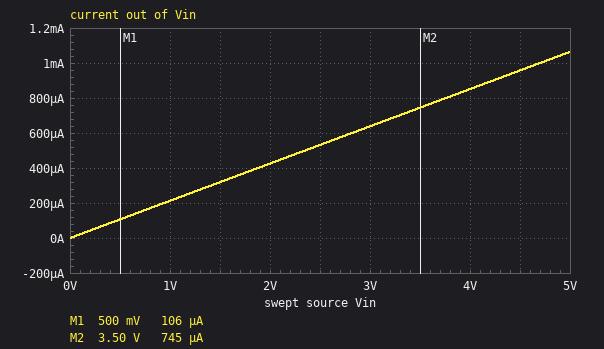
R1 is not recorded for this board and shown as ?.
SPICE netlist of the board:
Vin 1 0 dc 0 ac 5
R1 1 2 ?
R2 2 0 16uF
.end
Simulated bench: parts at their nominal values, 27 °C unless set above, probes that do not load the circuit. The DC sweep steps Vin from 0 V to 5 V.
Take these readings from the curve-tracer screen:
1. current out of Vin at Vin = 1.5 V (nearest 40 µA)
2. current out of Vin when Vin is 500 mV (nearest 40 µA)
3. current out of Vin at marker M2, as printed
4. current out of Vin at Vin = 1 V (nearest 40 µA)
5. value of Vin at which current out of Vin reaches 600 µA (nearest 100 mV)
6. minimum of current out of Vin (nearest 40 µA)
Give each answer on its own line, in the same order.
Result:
320 µA
120 µA
745 µA
200 µA
2.8 V
0 A
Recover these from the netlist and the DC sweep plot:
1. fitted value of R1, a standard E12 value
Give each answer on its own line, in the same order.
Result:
4.7 kΩ
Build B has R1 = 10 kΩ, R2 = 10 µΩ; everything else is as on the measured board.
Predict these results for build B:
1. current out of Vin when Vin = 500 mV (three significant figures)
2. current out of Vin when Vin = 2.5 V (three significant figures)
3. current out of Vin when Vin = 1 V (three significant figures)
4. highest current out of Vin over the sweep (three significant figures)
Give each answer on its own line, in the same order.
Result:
50.0 µA
250 µA
100 µA
500 µA
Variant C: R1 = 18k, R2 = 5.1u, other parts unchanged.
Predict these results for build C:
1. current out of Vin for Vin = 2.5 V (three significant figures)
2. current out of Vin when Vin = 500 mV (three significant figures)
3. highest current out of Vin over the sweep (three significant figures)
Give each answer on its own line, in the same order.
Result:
139 µA
27.8 µA
278 µA
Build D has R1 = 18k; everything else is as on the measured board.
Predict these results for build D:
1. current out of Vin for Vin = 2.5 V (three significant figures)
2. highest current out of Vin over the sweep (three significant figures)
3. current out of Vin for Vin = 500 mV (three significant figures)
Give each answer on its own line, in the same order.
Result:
139 µA
278 µA
27.8 µA
